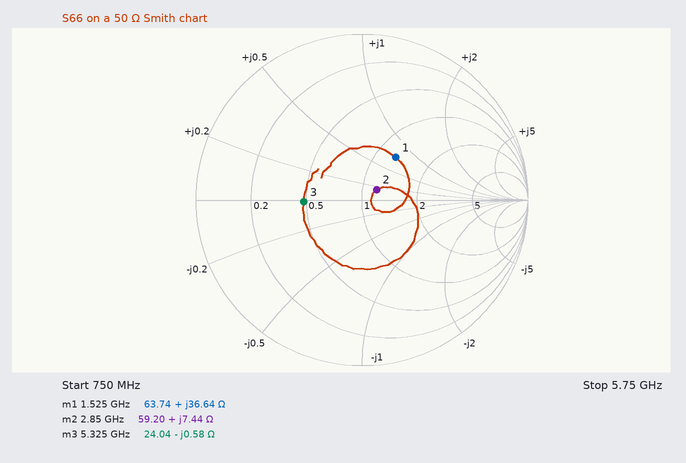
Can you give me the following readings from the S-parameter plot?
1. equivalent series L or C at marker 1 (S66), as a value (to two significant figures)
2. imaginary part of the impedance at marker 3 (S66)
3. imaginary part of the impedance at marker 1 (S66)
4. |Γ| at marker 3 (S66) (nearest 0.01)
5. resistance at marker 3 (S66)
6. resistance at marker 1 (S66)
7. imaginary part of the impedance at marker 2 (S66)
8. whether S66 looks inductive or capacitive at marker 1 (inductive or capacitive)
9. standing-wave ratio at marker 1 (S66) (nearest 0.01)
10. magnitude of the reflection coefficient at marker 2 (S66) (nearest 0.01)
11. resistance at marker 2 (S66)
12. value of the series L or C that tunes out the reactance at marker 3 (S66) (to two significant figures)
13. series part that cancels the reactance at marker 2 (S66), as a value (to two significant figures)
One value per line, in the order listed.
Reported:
3.8 nH
-0.58 Ω
+36.64 Ω
0.35
24.04 Ω
63.74 Ω
+7.44 Ω
inductive
1.97
0.11
59.20 Ω
17 pH
7.5 pF
